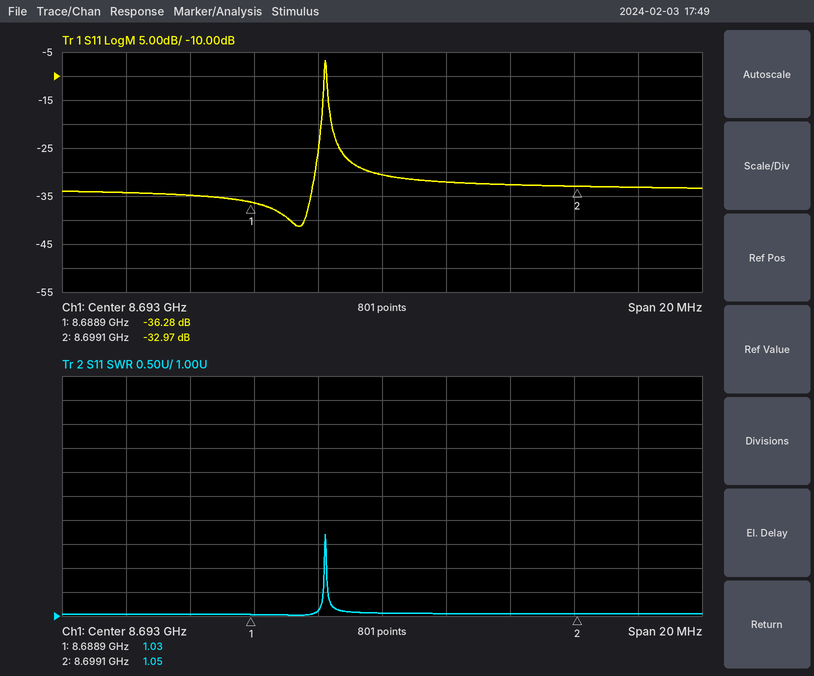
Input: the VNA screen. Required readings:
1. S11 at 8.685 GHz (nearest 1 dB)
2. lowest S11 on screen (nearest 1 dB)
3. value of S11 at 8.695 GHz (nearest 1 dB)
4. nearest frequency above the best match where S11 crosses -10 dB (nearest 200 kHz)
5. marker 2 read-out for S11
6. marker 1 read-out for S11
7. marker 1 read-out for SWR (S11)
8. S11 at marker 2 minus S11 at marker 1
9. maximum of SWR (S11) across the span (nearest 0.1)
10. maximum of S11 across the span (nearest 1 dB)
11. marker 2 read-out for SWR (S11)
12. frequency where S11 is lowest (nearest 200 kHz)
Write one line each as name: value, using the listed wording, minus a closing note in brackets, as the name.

S11 at 8.685 GHz: -34 dB
lowest S11 on screen: -41 dB
value of S11 at 8.695 GHz: -32 dB
nearest frequency above the best match where S11 crosses -10 dB: 8.6912 GHz
marker 2 read-out for S11: -32.97 dB
marker 1 read-out for S11: -36.28 dB
marker 1 read-out for SWR: 1.03
S11 at marker 2 minus S11 at marker 1: 3.31 dB
maximum of SWR (S11) across the span: 2.7
maximum of S11 across the span: -7 dB
marker 2 read-out for SWR: 1.05
frequency where S11 is lowest: 8.6904 GHz
